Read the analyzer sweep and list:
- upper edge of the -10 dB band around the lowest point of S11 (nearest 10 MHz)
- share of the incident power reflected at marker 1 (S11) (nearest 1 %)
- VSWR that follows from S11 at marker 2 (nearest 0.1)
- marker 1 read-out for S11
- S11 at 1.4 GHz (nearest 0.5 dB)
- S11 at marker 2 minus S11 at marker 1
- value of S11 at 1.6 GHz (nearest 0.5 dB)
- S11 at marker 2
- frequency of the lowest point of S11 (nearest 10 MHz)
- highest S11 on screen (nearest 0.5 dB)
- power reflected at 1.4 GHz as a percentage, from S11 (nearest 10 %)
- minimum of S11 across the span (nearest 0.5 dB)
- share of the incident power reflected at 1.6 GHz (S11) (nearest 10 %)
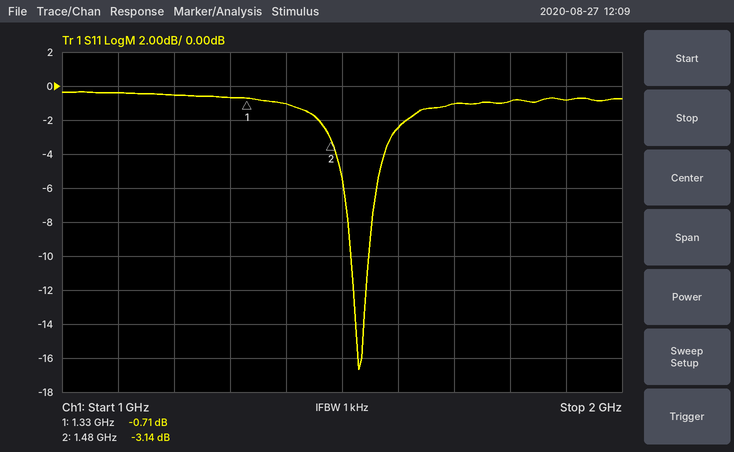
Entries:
1.55 GHz
85 %
5.6
-0.71 dB
-1.0 dB
-2.43 dB
-2.5 dB
-3.14 dB
1.53 GHz
-0.5 dB
80 %
-16.5 dB
60 %
